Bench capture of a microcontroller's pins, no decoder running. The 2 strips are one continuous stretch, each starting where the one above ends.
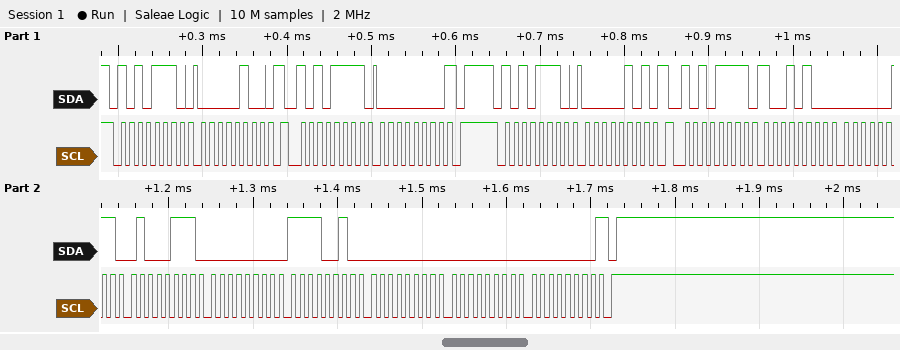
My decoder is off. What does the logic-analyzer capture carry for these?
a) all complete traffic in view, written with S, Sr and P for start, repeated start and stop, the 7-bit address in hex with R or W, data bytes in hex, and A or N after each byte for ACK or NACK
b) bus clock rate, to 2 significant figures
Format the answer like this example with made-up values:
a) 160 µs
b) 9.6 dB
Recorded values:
a) S 57W A 04 A Sr 57R A 00 N P S 57W A 05 A Sr 57R A 94 A 03 A 47 A 00 A F2 A 00 A 00 A 00 N P
b) 100 kHz
